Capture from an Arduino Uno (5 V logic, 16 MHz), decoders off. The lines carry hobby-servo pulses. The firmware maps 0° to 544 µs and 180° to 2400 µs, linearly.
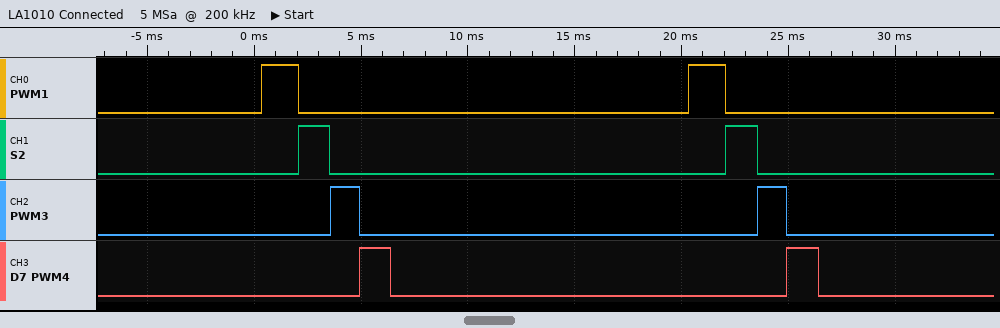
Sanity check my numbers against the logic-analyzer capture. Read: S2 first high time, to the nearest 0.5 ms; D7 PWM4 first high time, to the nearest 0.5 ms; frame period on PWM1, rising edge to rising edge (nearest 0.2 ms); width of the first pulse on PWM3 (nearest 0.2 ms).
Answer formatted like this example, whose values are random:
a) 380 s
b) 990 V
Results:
a) 1.5 ms
b) 1.5 ms
c) 20.0 ms
d) 1.4 ms
